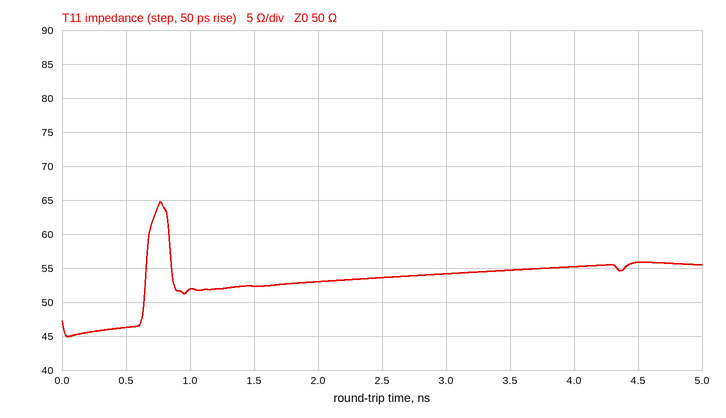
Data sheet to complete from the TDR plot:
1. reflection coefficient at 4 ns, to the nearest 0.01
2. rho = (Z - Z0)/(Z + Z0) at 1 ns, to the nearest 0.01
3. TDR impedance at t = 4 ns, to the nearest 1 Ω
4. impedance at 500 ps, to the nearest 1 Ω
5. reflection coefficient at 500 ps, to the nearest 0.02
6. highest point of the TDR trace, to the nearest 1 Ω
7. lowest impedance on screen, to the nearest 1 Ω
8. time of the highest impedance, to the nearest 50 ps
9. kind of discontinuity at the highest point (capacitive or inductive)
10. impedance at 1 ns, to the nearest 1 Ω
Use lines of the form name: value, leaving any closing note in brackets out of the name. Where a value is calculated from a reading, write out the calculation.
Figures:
reflection coefficient at 4 ns, to the nearest 0.01: (55 − 50)/(55 + 50) ≈ +0.05
rho = (Z - Z0)/(Z + Z0) at 1 ns, to the nearest 0.01: (52 − 50)/(52 + 50) ≈ +0.02
TDR impedance at t = 4 ns, to the nearest 1 Ω: 55 Ω
impedance at 500 ps, to the nearest 1 Ω: 46 Ω
reflection coefficient at 500 ps, to the nearest 0.02: (46 − 50)/(46 + 50) ≈ -0.04
highest point of the TDR trace, to the nearest 1 Ω: 65 Ω
lowest impedance on screen, to the nearest 1 Ω: 45 Ω
time of the highest impedance, to the nearest 50 ps: 750 ps
kind of discontinuity at the highest point: inductive
impedance at 1 ns, to the nearest 1 Ω: 52 Ω
